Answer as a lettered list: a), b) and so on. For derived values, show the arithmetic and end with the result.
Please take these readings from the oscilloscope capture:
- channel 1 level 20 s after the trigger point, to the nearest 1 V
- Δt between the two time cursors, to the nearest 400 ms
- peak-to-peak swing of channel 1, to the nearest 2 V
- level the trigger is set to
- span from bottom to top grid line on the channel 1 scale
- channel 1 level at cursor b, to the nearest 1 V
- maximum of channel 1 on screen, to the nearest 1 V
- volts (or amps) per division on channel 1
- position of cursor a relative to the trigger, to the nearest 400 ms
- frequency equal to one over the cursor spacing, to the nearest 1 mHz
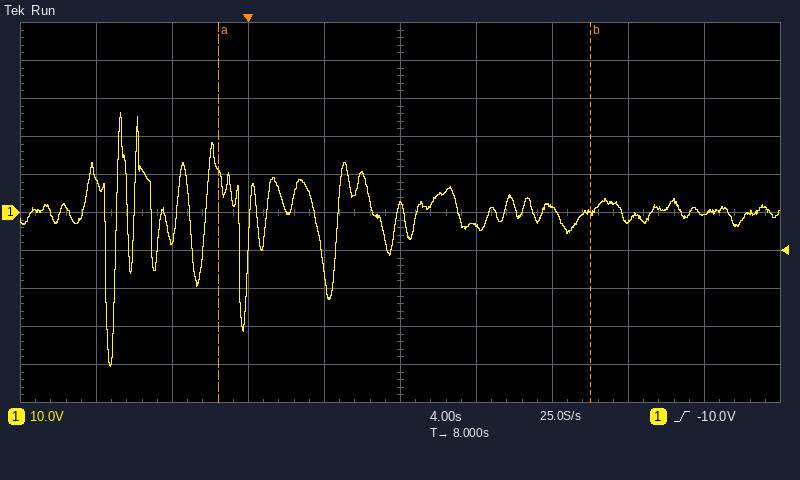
a) -2 V
b) 19.6 s
c) 66 V
d) -10.0 V
e) 100 V
f) 0 V
g) 26 V
h) 10 V
i) -1.6 s
j) 1 / 19.6 s ≈ 51 mHz
